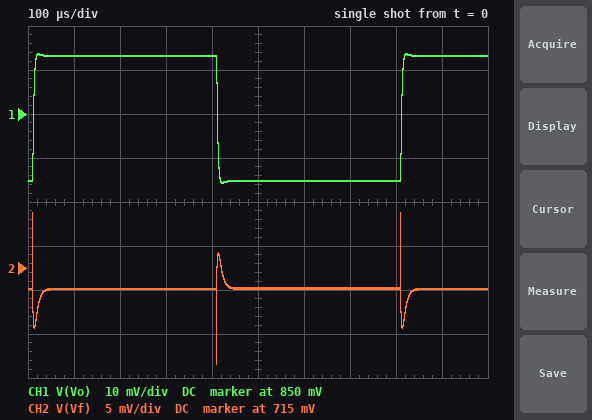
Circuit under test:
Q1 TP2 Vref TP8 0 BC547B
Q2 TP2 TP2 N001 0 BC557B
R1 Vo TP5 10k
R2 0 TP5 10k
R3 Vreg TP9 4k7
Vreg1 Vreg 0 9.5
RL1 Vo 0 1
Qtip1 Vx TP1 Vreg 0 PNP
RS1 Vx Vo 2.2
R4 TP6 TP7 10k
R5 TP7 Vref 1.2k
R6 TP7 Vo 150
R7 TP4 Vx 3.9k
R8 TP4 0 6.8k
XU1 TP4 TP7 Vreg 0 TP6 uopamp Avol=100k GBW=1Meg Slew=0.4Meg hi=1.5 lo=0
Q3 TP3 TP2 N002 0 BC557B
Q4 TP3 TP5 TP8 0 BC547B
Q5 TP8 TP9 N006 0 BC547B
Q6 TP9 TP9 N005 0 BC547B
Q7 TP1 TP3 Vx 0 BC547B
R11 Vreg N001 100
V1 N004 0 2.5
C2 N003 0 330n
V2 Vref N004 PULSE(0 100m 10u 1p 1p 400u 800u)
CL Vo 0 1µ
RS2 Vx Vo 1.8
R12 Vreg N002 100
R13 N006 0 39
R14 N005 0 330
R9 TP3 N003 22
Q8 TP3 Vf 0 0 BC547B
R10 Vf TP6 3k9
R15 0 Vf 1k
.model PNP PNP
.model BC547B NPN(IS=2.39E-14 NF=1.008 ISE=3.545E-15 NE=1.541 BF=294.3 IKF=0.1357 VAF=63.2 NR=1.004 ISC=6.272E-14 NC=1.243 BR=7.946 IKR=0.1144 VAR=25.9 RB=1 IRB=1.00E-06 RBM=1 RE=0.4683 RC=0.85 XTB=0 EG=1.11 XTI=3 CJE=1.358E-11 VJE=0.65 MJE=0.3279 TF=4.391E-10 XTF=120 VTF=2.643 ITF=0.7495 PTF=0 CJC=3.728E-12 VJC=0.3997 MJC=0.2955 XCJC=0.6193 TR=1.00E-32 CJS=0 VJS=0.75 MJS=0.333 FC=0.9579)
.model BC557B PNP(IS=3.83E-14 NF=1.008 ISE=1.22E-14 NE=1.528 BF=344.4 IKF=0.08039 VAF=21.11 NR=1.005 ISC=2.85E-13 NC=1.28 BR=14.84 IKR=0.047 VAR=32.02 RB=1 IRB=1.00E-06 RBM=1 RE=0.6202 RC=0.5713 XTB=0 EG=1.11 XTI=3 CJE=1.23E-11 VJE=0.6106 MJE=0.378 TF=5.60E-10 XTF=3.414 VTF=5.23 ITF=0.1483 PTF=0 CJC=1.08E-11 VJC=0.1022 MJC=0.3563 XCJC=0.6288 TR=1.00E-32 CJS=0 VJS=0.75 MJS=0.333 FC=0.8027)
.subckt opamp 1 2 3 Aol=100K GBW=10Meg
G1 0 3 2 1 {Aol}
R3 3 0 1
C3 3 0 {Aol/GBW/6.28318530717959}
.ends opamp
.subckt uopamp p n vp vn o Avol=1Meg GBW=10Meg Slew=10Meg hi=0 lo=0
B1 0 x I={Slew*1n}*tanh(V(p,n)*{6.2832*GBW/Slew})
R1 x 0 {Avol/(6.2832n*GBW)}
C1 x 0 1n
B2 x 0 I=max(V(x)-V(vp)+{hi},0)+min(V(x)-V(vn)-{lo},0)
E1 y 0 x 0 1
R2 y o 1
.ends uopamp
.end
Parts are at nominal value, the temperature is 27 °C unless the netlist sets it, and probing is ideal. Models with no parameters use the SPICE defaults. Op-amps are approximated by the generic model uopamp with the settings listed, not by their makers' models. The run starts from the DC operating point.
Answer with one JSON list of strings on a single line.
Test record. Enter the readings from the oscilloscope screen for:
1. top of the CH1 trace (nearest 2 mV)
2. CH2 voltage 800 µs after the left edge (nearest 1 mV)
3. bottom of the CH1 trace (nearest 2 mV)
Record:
["864 mV", "713 mV", "834 mV"]
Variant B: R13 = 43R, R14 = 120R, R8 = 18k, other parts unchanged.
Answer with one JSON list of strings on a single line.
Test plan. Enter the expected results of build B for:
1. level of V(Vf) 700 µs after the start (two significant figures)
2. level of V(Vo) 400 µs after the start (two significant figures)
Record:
["680 mV", "440 mV"]
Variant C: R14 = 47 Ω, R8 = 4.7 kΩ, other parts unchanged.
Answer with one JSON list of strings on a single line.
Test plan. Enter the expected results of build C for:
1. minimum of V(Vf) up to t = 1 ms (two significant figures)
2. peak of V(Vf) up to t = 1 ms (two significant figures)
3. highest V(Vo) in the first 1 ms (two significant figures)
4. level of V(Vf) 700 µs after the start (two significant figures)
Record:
["620 mV", "680 mV", "1.6 V", "660 mV"]
